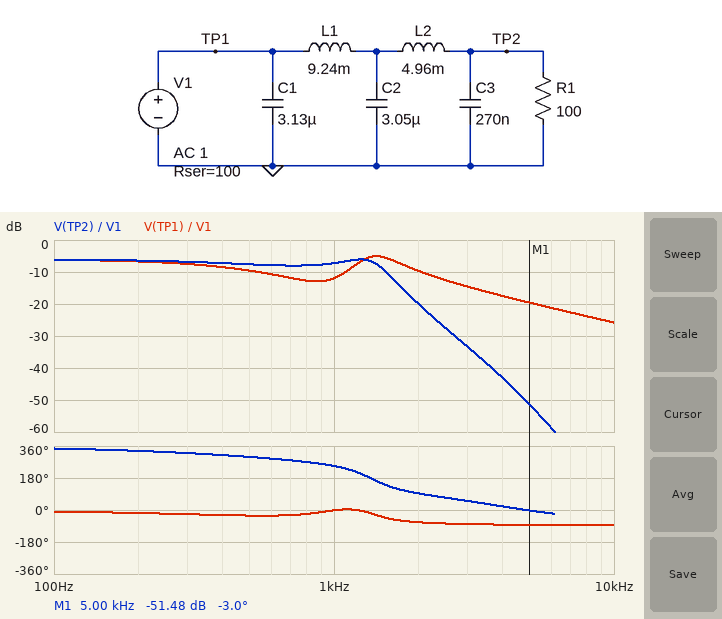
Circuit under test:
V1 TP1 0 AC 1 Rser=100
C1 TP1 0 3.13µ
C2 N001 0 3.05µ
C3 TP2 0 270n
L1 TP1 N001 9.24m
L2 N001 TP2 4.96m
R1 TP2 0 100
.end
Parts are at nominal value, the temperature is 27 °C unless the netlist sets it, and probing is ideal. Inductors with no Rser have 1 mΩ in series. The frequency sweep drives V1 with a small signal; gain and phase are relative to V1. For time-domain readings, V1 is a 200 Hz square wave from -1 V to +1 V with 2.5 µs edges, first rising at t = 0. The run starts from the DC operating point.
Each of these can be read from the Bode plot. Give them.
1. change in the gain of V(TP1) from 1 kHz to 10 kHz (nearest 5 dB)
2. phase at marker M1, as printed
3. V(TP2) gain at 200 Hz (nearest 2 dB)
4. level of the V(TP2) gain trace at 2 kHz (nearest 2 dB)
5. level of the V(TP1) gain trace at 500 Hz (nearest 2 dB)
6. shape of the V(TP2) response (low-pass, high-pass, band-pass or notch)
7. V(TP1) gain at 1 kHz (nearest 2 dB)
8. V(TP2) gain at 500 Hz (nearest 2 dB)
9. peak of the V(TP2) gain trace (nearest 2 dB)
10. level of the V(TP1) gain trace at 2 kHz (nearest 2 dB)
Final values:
-15 dB
-3.0 deg
-6 dB
-20 dB
-10 dB
low-pass
-12 dB
-8 dB
-6 dB
-10 dB
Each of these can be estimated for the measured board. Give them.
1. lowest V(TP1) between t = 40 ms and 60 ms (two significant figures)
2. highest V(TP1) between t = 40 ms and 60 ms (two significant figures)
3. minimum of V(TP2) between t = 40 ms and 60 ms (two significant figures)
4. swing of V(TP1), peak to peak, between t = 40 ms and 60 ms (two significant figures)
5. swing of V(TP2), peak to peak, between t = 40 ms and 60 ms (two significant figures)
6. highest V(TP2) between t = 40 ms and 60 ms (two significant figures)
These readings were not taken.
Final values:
-530 mV
530 mV
-530 mV
1.1 V
1.1 V
530 mV
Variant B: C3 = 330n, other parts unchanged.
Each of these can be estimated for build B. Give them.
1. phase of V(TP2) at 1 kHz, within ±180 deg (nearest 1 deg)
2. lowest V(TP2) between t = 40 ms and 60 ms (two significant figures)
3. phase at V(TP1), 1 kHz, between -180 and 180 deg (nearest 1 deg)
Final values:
-113 deg
-530 mV
-1 deg
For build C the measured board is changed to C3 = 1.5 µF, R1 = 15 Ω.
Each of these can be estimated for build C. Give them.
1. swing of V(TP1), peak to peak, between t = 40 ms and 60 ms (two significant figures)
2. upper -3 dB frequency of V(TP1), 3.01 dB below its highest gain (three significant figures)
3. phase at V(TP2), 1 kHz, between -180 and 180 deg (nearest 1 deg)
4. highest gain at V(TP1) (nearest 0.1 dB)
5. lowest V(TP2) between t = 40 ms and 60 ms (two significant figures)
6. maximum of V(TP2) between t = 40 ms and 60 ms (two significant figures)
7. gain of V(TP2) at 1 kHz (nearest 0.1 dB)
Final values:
1.3 V
1.13 kHz
-137 deg
-3.9 dB
-220 mV
220 mV
-16.8 dB
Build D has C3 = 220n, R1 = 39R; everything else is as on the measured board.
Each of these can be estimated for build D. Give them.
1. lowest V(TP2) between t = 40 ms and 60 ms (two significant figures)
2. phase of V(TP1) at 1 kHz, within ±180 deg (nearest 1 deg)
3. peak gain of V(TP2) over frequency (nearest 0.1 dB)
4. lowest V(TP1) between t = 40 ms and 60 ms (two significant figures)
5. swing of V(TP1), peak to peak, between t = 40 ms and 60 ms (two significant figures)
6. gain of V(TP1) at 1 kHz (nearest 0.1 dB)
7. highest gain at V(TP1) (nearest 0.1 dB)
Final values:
-380 mV
-25 deg
-10.3 dB
-510 mV
1.0 V
-8.0 dB
-7.4 dB
